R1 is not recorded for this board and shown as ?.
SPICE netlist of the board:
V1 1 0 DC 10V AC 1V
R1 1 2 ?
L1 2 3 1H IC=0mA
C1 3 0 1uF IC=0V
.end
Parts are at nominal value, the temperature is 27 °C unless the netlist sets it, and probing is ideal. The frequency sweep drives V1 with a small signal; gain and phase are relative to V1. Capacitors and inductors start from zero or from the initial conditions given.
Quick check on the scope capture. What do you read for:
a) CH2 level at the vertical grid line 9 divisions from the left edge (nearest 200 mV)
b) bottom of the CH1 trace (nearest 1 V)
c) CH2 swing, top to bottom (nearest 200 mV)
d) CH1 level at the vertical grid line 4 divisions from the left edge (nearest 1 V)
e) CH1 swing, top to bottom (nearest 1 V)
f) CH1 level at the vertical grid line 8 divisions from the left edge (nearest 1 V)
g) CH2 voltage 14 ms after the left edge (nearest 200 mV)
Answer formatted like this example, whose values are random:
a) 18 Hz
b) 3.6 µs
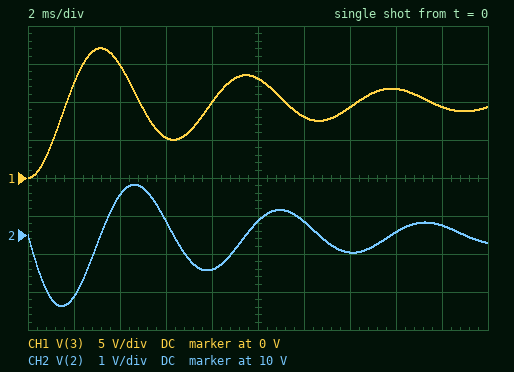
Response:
a) 10.2 V
b) 0 V
c) 3.2 V
d) 10 V
e) 17 V
f) 12 V
g) 9.6 V
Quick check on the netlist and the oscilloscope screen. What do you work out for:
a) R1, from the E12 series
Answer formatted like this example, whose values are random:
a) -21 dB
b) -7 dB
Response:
a) 220 Ω
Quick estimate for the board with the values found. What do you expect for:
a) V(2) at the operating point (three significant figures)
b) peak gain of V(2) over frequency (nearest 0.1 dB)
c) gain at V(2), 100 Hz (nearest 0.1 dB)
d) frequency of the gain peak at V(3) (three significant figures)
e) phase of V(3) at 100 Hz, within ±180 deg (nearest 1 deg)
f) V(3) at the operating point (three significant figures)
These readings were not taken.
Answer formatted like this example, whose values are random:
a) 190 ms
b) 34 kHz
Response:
a) 10.0 V
b) 0 dB
c) -0.2 dB
d) 157 Hz
e) -13 deg
f) 10.0 V
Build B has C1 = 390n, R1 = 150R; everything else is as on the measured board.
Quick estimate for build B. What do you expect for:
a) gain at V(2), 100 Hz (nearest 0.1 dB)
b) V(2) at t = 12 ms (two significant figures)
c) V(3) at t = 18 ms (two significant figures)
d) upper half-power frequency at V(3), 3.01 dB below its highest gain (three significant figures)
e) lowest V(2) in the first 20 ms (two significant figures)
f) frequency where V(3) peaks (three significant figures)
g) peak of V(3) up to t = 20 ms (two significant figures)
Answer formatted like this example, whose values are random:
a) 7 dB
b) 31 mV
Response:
a) 0 dB
b) 9.9 V
c) 12 V
d) 266 Hz
e) 9.1 V
f) 254 Hz
g) 19 V
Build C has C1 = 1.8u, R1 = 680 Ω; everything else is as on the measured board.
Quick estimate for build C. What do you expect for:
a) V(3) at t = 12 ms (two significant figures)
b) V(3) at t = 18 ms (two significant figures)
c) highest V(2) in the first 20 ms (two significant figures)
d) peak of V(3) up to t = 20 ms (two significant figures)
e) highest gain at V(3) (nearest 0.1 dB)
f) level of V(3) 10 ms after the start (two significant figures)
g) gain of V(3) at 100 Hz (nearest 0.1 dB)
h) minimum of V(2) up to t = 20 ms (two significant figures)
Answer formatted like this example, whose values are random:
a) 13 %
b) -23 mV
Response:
a) 9.9 V
b) 10 V
c) 11 V
d) 12 V
e) 1.8 dB
f) 9.6 V
g) 1.7 dB
h) 4.8 V
